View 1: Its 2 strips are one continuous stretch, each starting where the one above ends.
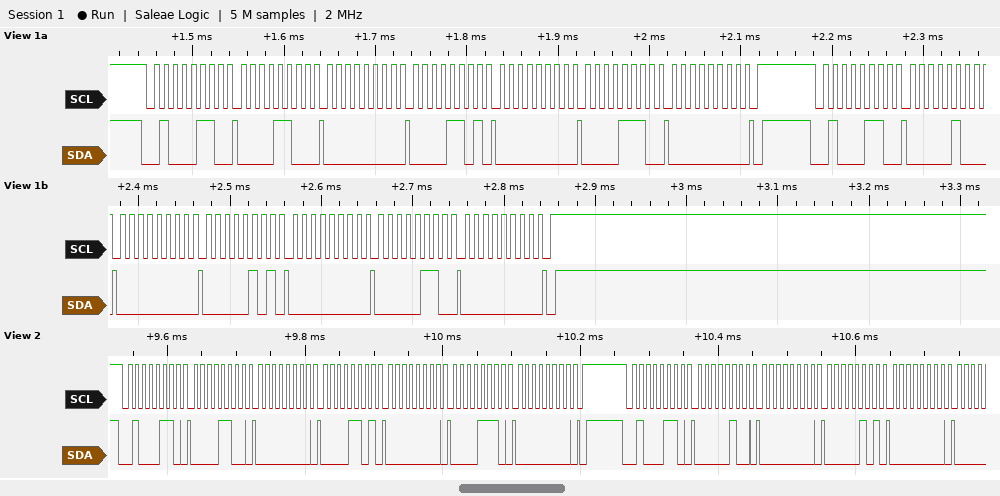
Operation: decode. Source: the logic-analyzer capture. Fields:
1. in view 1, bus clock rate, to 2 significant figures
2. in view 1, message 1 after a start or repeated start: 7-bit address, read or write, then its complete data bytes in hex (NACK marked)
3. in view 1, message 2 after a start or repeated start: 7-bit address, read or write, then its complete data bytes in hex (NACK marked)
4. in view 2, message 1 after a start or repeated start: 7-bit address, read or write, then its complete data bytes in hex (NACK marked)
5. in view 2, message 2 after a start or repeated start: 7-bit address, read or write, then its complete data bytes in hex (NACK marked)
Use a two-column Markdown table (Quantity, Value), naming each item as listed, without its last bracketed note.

| Quantity | Value |
|---|---|
| in view 1, bus clock rate, to 2 significant figures | 100 kHz |
| in view 1, message 1 after a start or repeated start: 7-bit address, read or write, then its complete data bytes in hex | 0x23 write: 0C 00 0D 00 0E 00 |
| in view 1, message 2 after a start or repeated start: 7-bit address, read or write, then its complete data bytes in hex | 0x23 write: 04 00 05 00 06 00 |
| in view 2, message 1 after a start or repeated start: 7-bit address, read or write, then its complete data bytes in hex | 0x23 write: 0C 00 0D 00 0E 00 |
| in view 2, message 2 after a start or repeated start: 7-bit address, read or write, then its complete data bytes in hex | 0x23 write: 04 00 05 00 |
